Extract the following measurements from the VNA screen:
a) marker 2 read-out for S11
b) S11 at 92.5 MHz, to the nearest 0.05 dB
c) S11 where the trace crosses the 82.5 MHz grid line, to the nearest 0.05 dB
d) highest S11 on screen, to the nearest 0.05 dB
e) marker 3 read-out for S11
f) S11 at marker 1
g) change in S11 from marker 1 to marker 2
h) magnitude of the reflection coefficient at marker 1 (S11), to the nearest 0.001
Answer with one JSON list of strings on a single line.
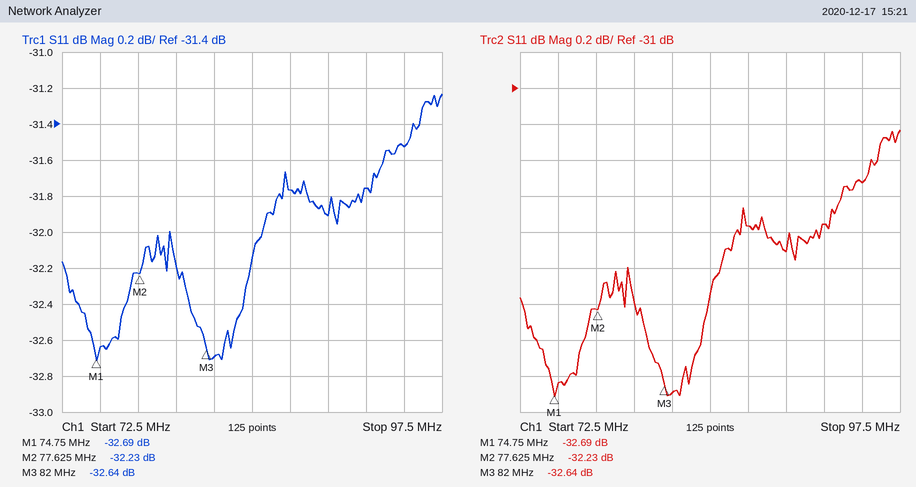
["-32.23 dB", "-31.75 dB", "-32.70 dB", "-31.25 dB", "-32.64 dB", "-32.69 dB", "0.46 dB", "0.023"]
